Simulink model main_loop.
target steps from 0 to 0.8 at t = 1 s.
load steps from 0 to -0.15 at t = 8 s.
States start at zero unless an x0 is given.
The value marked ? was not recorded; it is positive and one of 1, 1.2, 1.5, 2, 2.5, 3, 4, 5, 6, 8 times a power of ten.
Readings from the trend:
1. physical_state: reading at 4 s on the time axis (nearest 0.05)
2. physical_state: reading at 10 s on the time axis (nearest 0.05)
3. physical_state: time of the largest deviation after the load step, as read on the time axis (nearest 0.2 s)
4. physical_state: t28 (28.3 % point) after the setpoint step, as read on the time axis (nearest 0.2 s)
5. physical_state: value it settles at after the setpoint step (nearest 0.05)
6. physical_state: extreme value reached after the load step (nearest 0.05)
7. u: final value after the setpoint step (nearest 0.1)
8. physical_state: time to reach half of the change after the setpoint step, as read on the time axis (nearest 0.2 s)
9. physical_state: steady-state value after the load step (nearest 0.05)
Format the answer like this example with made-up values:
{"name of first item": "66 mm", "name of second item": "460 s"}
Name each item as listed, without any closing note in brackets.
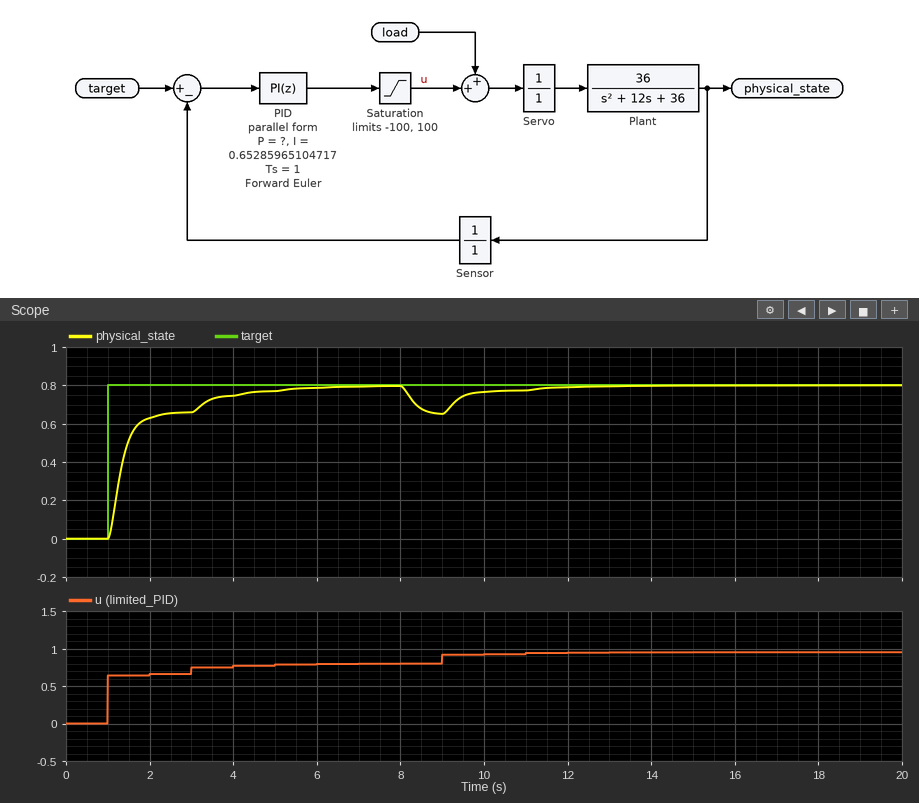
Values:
{"physical_state: reading at 4 s on the time axis": "0.75", "physical_state: reading at 10 s on the time axis": "0.75", "physical_state: time of the largest deviation after the load step, as read on the time axis": "9.0 s", "physical_state: t28 (28.3 % point) after the setpoint step, as read on the time axis": "1.2 s", "physical_state: value it settles at after the setpoint step": "0.80", "physical_state: extreme value reached after the load step": "0.65", "u: final value after the setpoint step": "0.8", "physical_state: time to reach half of the change after the setpoint step, as read on the time axis": "1.4 s", "physical_state: steady-state value after the load step": "0.80"}
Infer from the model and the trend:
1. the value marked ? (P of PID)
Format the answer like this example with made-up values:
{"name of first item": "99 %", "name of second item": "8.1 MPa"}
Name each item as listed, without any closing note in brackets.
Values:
{"the value marked ?": "0.8"}
